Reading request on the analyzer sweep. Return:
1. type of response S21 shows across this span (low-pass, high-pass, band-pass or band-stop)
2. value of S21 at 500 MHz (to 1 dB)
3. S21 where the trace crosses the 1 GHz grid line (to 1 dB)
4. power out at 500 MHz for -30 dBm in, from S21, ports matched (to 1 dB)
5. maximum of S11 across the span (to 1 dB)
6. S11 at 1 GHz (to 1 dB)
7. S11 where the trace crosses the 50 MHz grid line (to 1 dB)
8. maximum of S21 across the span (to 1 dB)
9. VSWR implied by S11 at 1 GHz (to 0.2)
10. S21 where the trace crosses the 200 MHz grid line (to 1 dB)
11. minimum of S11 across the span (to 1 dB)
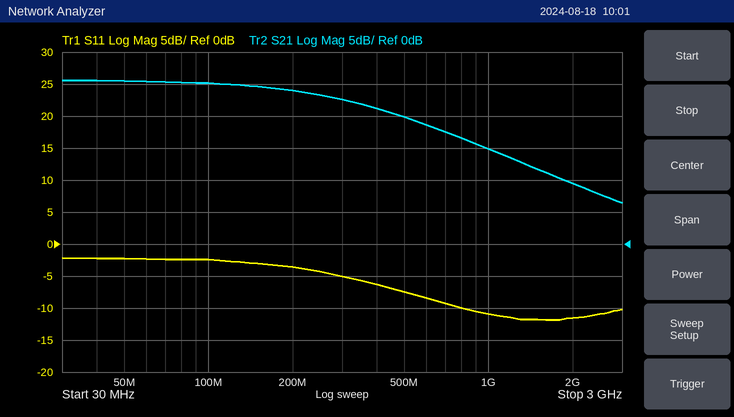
low-pass
20 dB
15 dB
-10 dBm
-2 dB
-11 dB
-2 dB
26 dB
1.8
24 dB
-12 dB
